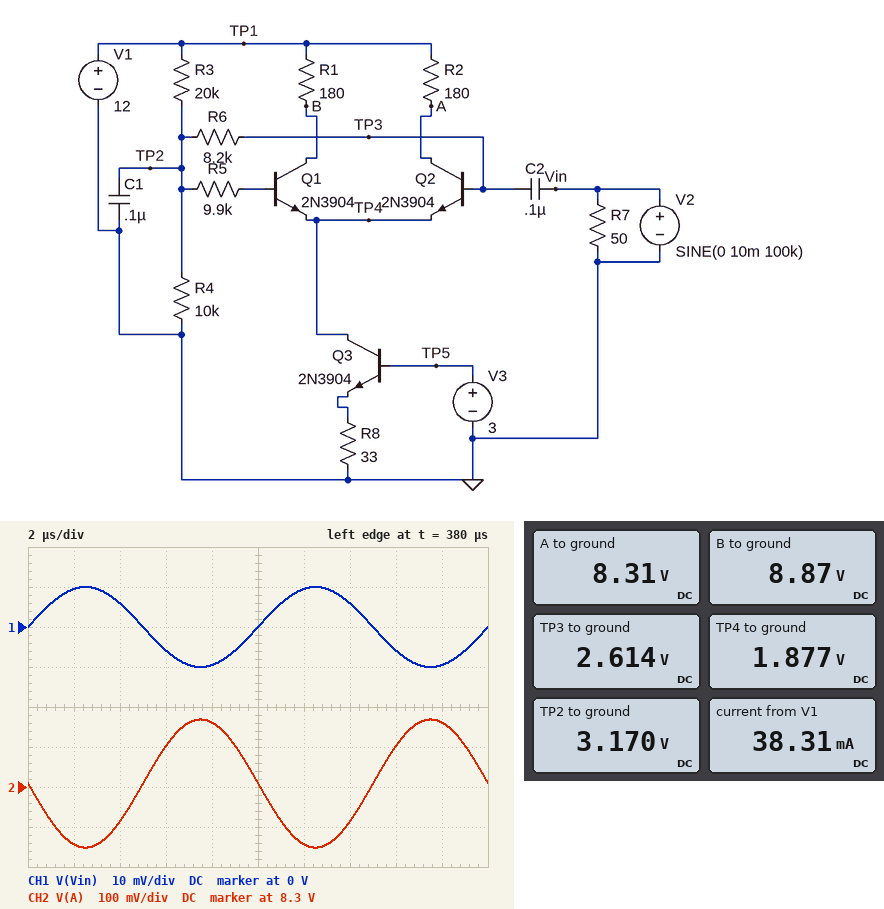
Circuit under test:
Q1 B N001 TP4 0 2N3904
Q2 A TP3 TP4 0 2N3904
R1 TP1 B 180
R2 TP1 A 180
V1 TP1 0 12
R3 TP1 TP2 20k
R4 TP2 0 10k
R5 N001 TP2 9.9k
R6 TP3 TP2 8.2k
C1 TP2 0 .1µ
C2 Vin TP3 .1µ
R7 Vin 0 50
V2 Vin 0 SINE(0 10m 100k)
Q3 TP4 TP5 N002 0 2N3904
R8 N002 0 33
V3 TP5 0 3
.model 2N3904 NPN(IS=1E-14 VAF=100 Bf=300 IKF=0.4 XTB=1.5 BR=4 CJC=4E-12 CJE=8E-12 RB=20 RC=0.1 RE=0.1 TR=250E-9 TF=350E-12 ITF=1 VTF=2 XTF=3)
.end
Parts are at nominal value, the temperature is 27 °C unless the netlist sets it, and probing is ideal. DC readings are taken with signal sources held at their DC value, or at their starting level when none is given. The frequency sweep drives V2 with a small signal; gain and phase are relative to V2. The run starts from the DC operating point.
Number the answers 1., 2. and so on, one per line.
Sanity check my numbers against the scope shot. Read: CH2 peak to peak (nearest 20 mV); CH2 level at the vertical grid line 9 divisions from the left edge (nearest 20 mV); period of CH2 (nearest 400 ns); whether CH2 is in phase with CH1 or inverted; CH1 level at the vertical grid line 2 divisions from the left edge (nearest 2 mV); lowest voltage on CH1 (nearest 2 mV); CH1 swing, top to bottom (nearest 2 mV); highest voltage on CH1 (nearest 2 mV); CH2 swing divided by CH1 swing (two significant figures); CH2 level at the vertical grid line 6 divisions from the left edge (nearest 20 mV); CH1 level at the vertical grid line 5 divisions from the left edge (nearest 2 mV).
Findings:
1. 320 mV
2. 8.46 V
3. 10.0 µs
4. inverted
5. 6 mV
6. -10 mV
7. 20 mV
8. 10 mV
9. 16
10. 8.16 V
11. 0 V
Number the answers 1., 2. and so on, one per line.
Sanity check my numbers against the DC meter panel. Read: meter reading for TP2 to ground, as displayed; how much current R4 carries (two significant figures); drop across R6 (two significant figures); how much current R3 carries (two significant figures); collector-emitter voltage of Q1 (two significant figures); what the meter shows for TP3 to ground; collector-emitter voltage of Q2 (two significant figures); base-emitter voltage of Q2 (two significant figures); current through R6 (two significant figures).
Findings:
1. 3.170 V
2. 320 µA
3. 560 mV
4. 440 µA
5. 7.0 V
6. 2.614 V
7. 6.4 V
8. 740 mV
9. 68 µA
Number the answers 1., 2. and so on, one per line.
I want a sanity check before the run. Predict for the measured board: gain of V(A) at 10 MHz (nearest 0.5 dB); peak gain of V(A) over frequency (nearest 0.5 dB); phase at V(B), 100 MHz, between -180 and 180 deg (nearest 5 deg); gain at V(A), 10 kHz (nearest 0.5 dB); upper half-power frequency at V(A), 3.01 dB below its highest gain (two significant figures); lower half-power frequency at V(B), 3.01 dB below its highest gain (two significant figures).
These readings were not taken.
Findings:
1. 22.5 dB
2. 24.0 dB
3. -25 deg
4. 24.0 dB
5. 57 MHz
6. 1.0 kHz
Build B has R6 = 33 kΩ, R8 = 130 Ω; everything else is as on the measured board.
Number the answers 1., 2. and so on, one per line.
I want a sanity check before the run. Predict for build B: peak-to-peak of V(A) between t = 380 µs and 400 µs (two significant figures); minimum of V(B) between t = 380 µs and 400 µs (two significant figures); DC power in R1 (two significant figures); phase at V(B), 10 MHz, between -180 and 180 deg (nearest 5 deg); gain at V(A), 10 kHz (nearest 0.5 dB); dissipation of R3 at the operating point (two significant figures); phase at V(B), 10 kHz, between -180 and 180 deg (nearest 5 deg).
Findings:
1. 85 mV
2. 9.6 V
3. 30 mW
4. -35 deg
5. 12.5 dB
6. 3.5 mW
7. 0 deg
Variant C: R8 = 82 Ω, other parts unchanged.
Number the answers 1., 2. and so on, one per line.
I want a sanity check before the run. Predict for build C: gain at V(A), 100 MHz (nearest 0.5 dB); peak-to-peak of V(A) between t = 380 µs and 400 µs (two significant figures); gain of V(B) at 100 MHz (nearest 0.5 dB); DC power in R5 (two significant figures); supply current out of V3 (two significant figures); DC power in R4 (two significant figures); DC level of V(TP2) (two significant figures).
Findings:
1. 18.0 dB
2. 150 mV
3. -9.5 dB
4. 15 µW
5. 600 µA
6. 1.2 mW
7. 3.4 V
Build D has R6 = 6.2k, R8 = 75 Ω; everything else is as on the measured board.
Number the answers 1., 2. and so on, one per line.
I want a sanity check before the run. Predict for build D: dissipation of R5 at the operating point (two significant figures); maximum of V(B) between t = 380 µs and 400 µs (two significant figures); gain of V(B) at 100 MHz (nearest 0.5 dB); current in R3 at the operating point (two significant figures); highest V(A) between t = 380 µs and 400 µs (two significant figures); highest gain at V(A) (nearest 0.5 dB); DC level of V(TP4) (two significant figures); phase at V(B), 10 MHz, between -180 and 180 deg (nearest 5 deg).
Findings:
1. 13 µW
2. 10 V
3. -9.5 dB
4. 430 µA
5. 9.0 V
6. 21.0 dB
7. 2.3 V
8. -40 deg
